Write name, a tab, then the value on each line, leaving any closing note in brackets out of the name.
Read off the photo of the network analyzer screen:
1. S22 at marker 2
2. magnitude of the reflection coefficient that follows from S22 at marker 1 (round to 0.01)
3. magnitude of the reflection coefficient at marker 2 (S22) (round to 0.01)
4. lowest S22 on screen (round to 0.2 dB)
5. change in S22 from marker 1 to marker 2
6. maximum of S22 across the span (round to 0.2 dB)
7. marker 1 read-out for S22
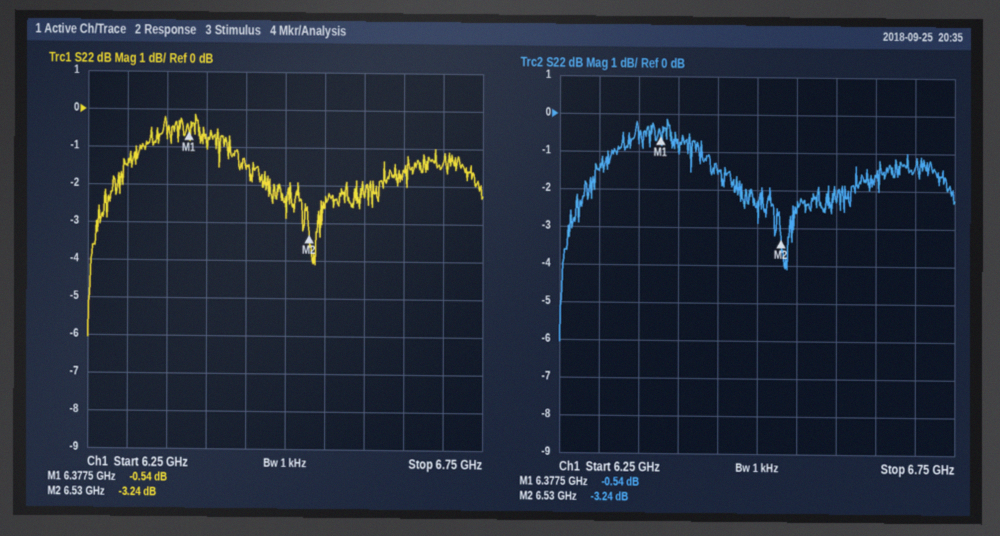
S22 at marker 2	-3.24 dB
magnitude of the reflection coefficient that follows from S22 at marker 1	0.94
magnitude of the reflection coefficient at marker 2 (S22)	0.69
lowest S22 on screen	-6.0 dB
change in S22 from marker 1 to marker 2	-2.70 dB
maximum of S22 across the span	-0.2 dB
marker 1 read-out for S22	-0.54 dB
